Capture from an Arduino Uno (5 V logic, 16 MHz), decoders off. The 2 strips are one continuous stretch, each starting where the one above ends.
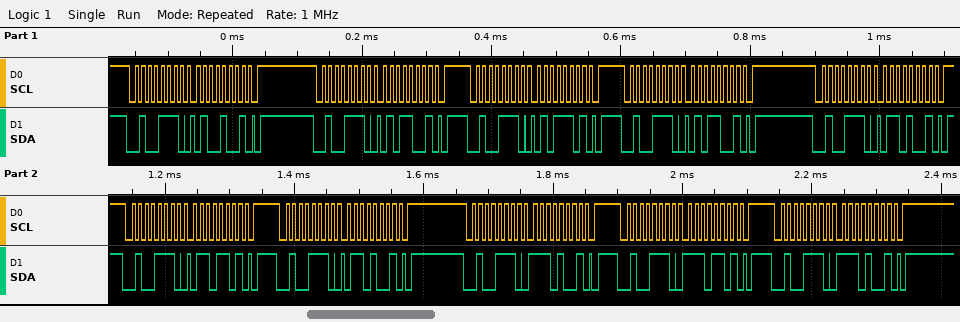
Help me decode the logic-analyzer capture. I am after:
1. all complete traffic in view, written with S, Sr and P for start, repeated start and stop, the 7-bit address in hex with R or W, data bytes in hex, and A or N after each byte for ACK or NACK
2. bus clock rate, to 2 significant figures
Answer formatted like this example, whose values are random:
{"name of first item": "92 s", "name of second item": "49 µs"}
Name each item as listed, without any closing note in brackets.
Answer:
{"all complete traffic in view, written with S, Sr and P for start, repeated start and stop, the 7-bit address in hex with R or W, data bytes in hex, and A or N after each byte for ACK or NACK": "S 27W A 49 A P S 27W A 59 A P S 27W A 5D A P S 27W A 59 A P S 27W A 69 A P S 27W A 6D A P S 27W A 69 A P S 27W A E9 A P S 27W A ED A P S 27W A E9 A P", "bus clock rate, to 2 significant figures": "100 kHz"}
